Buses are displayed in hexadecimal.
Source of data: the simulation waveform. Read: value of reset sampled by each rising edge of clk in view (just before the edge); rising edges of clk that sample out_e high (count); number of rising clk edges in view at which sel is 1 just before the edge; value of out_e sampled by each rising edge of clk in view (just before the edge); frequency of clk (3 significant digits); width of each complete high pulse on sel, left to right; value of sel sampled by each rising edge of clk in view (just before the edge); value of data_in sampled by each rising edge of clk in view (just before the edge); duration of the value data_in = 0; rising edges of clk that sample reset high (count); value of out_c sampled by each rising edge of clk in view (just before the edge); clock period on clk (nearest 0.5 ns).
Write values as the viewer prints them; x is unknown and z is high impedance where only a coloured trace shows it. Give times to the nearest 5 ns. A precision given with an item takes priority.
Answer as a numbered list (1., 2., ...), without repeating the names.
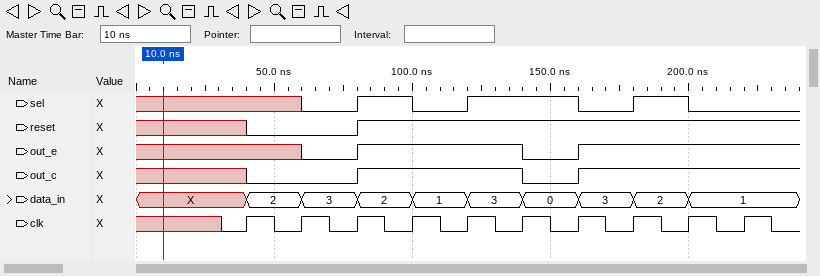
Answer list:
1. x 0 0 1 1 1 1 1 1 1
2. 6
3. 4
4. x x 0 1 1 1 0 1 1 1
5. 50.0 MHz
6. 20 ns, 40 ns, 20 ns
7. x x 0 1 0 1 1 0 1 0
8. X, 2, 3, 2, 1, 3, 0, 3, 2, 1
9. 20 ns
10. 7
11. x 0 0 1 1 1 0 1 1 1
12. 20 ns
